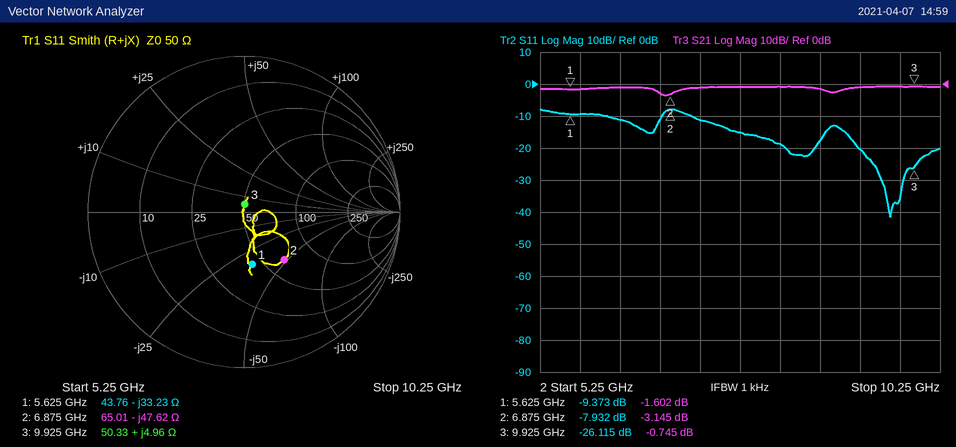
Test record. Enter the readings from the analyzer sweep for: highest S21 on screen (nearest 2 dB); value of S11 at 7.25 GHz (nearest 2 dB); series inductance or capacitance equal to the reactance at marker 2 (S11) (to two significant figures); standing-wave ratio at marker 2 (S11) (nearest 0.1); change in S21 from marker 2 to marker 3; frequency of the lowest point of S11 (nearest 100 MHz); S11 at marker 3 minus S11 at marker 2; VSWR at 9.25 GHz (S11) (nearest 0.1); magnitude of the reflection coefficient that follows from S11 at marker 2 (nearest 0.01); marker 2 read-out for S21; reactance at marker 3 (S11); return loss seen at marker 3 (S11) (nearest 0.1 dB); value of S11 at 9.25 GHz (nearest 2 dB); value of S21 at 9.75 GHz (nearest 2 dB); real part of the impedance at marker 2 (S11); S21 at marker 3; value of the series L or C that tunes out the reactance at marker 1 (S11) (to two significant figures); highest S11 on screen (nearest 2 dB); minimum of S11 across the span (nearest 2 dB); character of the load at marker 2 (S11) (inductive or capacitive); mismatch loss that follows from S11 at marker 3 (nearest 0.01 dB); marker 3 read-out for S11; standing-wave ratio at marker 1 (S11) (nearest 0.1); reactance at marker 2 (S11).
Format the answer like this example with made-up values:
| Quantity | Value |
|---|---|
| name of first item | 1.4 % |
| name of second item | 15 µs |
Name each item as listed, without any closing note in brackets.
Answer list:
| Quantity | Value |
|---|---|
| highest S21 on screen | 0 dB |
| value of S11 at 7.25 GHz | -12 dB |
| series inductance or capacitance equal to the reactance at marker 2 (S11) | 490 fF |
| standing-wave ratio at marker 2 (S11) | 2.3 |
| change in S21 from marker 2 to marker 3 | 2.400 dB |
| frequency of the lowest point of S11 | 9.6 GHz |
| S11 at marker 3 minus S11 at marker 2 | -18.183 dB |
| VSWR at 9.25 GHz (S11) | 1.2 |
| magnitude of the reflection coefficient that follows from S11 at marker 2 | 0.40 |
| marker 2 read-out for S21 | -3.145 dB |
| reactance at marker 3 | +4.96 Ω |
| return loss seen at marker 3 (S11) | 26.1 dB |
| value of S11 at 9.25 GHz | -20 dB |
| value of S21 at 9.75 GHz | 0 dB |
| real part of the impedance at marker 2 | 65.01 Ω |
| S21 at marker 3 | -0.745 dB |
| value of the series L or C that tunes out the reactance at marker 1 (S11) | 940 pH |
| highest S11 on screen | -8 dB |
| minimum of S11 across the span | -42 dB |
| character of the load at marker 2 (S11) | capacitive |
| mismatch loss that follows from S11 at marker 3 | 0.01 dB |
| marker 3 read-out for S11 | -26.115 dB |
| standing-wave ratio at marker 1 (S11) | 2.0 |
| reactance at marker 2 | -47.62 Ω |
